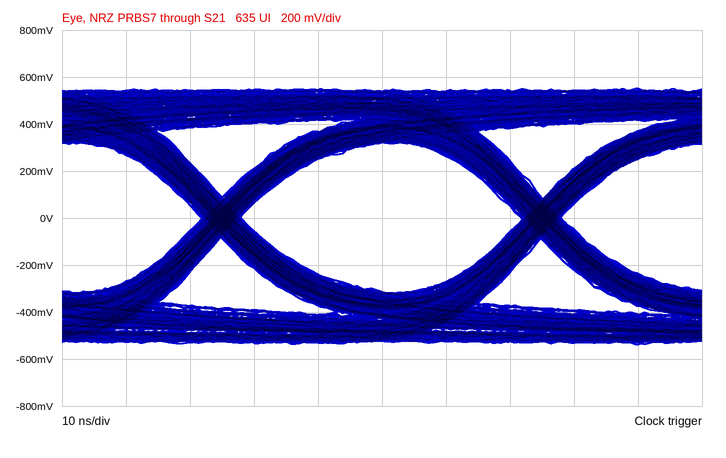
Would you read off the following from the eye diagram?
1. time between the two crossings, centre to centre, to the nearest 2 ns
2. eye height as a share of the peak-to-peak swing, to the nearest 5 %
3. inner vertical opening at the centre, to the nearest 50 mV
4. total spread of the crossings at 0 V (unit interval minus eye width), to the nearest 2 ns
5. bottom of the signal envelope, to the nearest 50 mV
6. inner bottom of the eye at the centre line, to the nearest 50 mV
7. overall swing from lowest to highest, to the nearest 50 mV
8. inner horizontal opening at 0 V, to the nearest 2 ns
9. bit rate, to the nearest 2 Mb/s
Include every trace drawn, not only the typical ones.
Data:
50 ns
60 %
650 mV
6 ns
-550 mV
-300 mV
1.10 V
44 ns
20 Mb/s
